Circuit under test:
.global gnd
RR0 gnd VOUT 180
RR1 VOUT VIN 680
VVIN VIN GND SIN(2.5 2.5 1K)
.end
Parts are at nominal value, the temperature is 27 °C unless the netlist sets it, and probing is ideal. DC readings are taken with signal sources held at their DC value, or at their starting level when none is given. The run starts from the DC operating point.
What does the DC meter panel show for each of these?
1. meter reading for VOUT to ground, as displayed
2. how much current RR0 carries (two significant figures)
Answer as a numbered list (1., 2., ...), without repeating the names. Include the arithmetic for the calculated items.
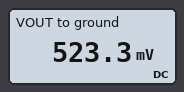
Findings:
1. 523.3 mV
2. (523.3 mV) / 180 Ω = 2.9 mA
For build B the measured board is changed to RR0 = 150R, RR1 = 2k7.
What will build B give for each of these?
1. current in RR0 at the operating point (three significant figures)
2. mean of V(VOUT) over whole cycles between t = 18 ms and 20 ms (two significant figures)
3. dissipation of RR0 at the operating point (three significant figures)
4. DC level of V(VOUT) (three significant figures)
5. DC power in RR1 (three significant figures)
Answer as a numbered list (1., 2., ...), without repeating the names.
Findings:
1. 877 µA
2. 130 mV
3. 115 µW
4. 132 mV
5. 2.08 mW
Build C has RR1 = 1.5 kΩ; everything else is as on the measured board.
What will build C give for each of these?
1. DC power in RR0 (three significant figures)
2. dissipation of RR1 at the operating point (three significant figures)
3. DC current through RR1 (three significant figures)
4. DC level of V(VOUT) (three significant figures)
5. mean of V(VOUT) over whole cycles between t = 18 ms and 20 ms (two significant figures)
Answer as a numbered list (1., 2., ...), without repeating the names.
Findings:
1. 399 µW
2. 3.32 mW
3. 1.49 mA
4. 268 mV
5. 270 mV
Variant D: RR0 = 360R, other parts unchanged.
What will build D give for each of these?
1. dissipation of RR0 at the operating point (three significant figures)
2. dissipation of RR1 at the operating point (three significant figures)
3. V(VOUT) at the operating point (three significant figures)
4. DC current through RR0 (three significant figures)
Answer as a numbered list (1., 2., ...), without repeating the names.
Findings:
1. 2.08 mW
2. 3.93 mW
3. 865 mV
4. 2.40 mA
